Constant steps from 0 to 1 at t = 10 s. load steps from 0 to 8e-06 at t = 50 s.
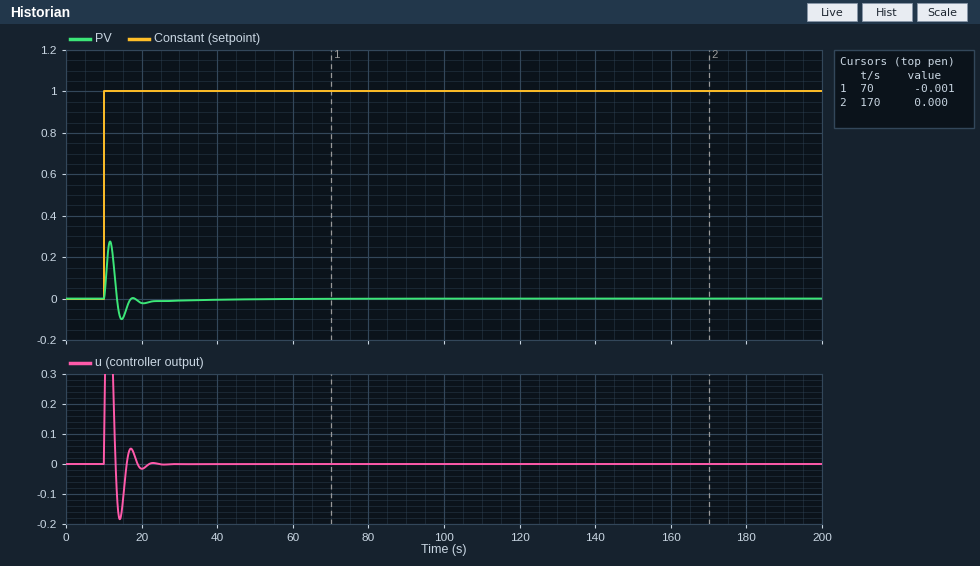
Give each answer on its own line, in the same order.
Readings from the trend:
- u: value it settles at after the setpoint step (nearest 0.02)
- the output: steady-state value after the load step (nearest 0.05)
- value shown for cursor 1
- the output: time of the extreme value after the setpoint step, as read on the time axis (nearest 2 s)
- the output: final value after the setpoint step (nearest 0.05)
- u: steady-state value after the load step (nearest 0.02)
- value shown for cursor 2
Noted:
0.00
0.00
-0.001
12 s
0.00
0.00
0.000
